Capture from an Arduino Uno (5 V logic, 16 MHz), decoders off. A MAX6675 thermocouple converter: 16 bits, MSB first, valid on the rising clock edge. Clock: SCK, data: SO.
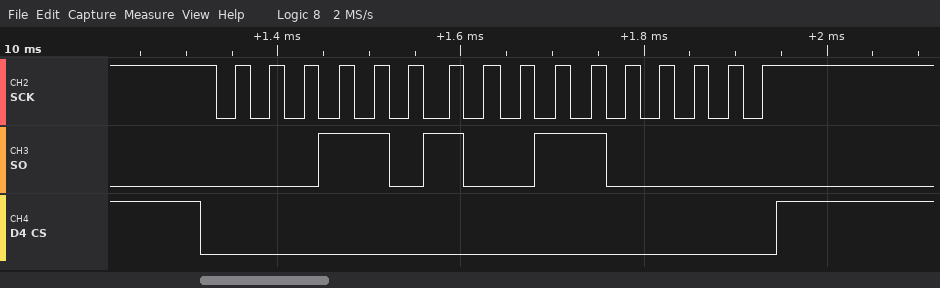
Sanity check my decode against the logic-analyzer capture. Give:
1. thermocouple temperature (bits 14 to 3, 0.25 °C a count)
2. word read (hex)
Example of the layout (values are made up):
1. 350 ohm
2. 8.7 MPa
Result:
1. 211.00 °C
2. 0x1A60
